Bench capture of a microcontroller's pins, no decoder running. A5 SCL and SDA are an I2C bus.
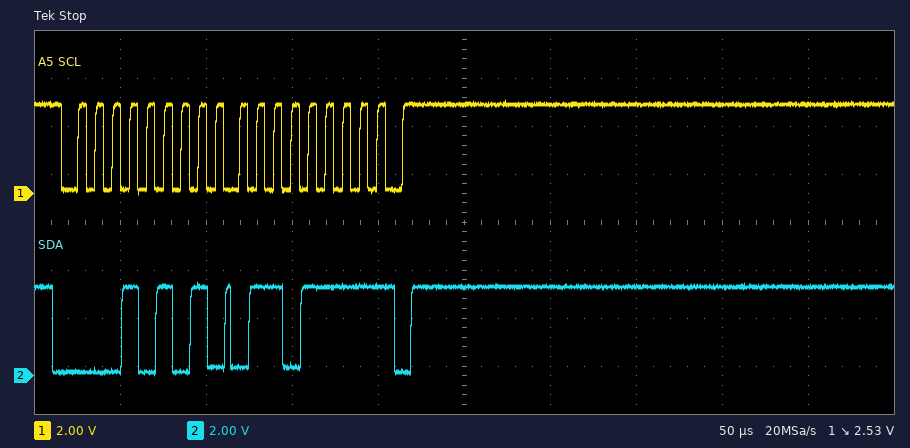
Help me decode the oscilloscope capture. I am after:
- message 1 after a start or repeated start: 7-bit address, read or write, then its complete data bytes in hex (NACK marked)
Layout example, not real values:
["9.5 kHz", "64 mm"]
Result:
["0x0A read: 6F NACK"]
